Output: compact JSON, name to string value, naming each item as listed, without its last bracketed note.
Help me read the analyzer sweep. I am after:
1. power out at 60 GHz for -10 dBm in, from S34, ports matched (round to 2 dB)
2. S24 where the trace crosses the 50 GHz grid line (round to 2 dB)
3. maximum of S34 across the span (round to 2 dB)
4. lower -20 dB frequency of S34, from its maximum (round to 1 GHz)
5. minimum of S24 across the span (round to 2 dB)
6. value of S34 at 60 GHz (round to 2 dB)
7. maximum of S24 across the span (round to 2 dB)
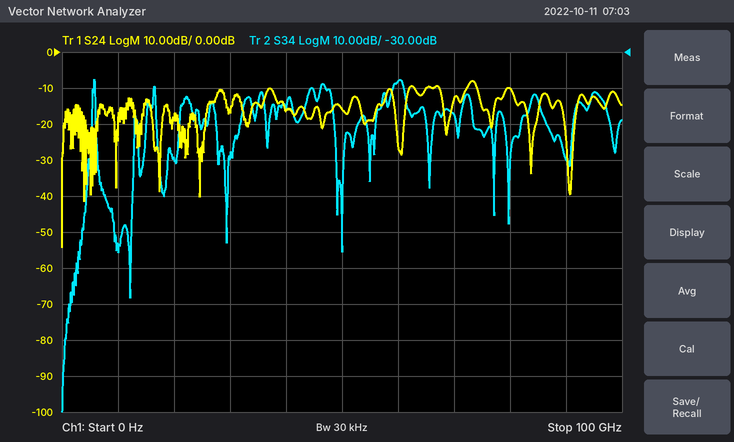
{"power out at 60 GHz for -10 dBm in, from S34, ports matched": "-48 dBm", "S24 where the trace crosses the 50 GHz grid line": "-16 dB", "maximum of S34 across the span": "-38 dB", "lower -20 dB frequency of S34, from its maximum": "5 GHz", "minimum of S24 across the span": "-54 dB", "value of S34 at 60 GHz": "-38 dB", "maximum of S24 across the span": "-8 dB"}
